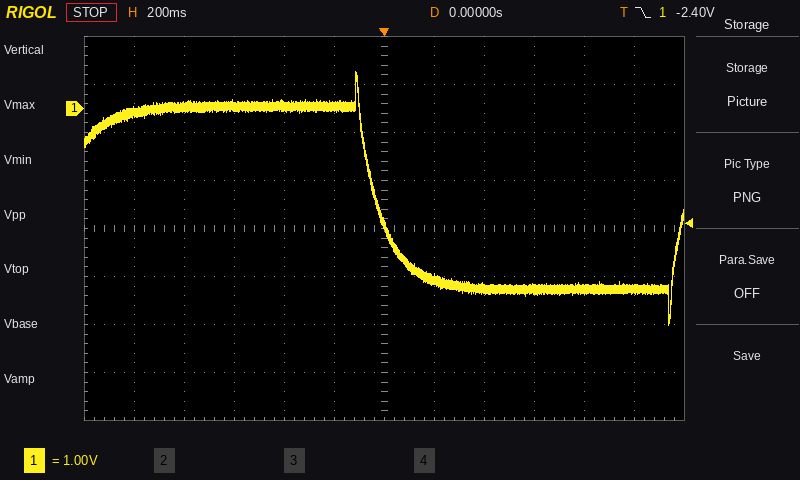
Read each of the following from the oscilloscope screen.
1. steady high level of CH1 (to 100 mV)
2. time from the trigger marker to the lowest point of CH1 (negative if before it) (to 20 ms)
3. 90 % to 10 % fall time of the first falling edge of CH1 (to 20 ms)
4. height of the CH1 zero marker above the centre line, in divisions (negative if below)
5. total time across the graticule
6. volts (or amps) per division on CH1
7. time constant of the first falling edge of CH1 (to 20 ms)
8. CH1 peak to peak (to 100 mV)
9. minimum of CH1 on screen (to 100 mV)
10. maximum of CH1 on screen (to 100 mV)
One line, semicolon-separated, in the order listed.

0.0 V; +1.14 s; 220 ms; +2.5 div; 2.4 s; 1 V; 100 ms; 5.3 V; -4.5 V; 800 mV
